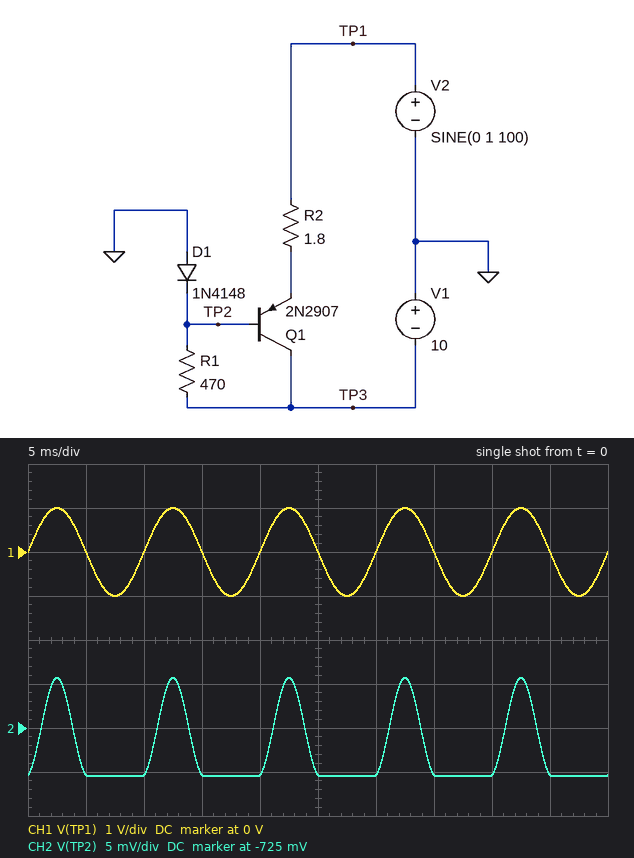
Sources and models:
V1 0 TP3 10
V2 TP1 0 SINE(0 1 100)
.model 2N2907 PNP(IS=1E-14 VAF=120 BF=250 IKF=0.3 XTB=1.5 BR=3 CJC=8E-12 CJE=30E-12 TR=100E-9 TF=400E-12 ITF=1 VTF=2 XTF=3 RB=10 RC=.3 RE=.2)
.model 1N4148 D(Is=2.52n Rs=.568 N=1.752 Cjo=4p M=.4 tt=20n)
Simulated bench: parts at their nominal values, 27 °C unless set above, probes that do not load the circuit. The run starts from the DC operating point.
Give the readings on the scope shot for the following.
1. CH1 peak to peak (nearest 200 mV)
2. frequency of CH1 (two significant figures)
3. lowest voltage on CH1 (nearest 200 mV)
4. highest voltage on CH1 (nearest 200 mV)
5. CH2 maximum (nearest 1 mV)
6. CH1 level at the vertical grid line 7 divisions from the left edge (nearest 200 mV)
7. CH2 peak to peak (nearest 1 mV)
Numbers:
2.0 V
100 Hz
-1.0 V
1.0 V
-719 mV
0 V
11 mV
